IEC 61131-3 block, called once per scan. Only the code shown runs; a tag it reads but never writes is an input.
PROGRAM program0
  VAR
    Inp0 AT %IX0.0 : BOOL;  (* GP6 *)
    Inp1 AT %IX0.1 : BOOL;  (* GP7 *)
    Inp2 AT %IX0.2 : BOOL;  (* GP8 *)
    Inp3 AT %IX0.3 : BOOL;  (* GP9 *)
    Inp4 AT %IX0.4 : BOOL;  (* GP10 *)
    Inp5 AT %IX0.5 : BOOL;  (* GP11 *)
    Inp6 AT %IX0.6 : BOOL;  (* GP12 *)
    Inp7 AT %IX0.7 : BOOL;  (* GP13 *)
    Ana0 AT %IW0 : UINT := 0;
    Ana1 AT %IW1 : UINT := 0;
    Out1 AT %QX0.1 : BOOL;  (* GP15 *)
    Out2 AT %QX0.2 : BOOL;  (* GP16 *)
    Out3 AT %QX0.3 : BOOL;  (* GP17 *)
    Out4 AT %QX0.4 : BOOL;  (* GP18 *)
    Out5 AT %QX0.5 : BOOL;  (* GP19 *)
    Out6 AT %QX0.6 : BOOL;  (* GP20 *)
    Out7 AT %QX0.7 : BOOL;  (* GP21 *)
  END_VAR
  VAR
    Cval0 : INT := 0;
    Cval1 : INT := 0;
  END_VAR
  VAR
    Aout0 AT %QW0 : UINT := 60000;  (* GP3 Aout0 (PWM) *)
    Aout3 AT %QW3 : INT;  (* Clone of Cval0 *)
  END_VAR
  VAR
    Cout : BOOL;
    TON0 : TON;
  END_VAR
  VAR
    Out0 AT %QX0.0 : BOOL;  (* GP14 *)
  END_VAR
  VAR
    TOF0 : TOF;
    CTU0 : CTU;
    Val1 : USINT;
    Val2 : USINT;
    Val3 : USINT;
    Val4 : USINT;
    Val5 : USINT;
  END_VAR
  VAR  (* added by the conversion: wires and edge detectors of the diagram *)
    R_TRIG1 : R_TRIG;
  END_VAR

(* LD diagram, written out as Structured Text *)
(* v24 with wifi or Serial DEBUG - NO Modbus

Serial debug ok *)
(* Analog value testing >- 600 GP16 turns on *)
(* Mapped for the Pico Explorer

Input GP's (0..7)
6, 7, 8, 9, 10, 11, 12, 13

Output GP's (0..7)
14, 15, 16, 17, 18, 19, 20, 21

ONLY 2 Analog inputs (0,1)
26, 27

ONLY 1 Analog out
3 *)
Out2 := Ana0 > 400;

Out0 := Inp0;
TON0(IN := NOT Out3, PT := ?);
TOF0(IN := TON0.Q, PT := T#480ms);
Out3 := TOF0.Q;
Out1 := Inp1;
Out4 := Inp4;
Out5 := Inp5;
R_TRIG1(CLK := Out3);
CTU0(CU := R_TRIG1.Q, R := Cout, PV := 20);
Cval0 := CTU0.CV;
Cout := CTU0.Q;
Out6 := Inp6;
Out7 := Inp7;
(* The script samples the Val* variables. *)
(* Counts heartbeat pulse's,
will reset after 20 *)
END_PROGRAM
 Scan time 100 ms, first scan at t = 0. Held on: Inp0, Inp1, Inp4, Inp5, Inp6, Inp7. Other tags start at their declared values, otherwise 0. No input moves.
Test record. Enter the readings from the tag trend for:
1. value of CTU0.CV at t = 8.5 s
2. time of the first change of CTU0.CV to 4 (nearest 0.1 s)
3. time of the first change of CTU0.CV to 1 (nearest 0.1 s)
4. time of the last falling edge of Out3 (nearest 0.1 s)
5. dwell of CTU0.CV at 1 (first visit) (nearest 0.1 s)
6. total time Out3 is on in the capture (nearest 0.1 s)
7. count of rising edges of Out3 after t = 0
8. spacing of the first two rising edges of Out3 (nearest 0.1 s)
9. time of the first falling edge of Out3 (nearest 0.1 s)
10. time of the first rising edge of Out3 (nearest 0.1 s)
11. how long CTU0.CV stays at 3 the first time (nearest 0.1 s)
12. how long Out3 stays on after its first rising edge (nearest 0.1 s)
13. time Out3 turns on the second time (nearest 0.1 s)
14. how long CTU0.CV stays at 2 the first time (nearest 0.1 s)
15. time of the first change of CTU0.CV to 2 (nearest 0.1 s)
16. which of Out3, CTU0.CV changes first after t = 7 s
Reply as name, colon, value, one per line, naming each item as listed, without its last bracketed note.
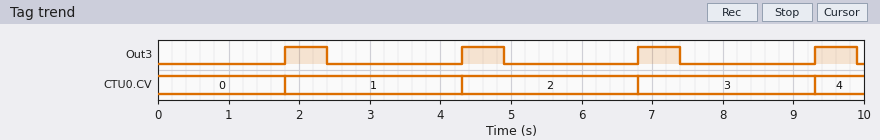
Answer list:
value of CTU0.CV at t = 8.5 s: 3
time of the first change of CTU0.CV to 4: 9.3 s
time of the first change of CTU0.CV to 1: 1.8 s
time of the last falling edge of Out3: 9.9 s
dwell of CTU0.CV at 1 (first visit): 2.5 s
total time Out3 is on in the capture: 2.4 s
count of rising edges of Out3 after t = 0: 4
spacing of the first two rising edges of Out3: 2.5 s
time of the first falling edge of Out3: 2.4 s
time of the first rising edge of Out3: 1.8 s
how long CTU0.CV stays at 3 the first time: 2.5 s
how long Out3 stays on after its first rising edge: 0.6 s
time Out3 turns on the second time: 4.3 s
how long CTU0.CV stays at 2 the first time: 2.5 s
time of the first change of CTU0.CV to 2: 4.3 s
which of Out3, CTU0.CV changes first after t = 7 s: Out3
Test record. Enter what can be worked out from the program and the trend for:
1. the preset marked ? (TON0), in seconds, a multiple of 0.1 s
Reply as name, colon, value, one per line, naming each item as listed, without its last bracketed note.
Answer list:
the preset marked ? (TON0), in seconds, a multiple of 0.1 s: 1.8 s
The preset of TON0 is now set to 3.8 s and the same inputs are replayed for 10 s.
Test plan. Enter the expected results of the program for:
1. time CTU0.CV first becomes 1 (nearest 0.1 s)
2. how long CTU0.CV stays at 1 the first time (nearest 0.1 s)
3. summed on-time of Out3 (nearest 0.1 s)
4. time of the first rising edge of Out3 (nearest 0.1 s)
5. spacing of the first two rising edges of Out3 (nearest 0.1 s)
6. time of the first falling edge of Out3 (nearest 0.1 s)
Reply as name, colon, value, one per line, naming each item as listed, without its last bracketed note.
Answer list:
time CTU0.CV first becomes 1: 3.8 s
how long CTU0.CV stays at 1 the first time: 4.5 s
summed on-time of Out3: 1.2 s
time of the first rising edge of Out3: 3.8 s
spacing of the first two rising edges of Out3: 4.5 s
time of the first falling edge of Out3: 4.4 s
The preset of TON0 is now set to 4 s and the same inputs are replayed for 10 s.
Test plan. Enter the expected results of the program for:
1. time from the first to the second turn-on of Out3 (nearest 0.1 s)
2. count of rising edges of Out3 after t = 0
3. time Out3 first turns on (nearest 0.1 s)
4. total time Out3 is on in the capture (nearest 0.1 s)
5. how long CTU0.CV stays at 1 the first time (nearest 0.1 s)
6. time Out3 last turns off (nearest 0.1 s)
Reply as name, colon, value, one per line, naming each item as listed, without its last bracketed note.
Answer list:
time from the first to the second turn-on of Out3: 4.7 s
count of rising edges of Out3 after t = 0: 2
time Out3 first turns on: 4.0 s
total time Out3 is on in the capture: 1.2 s
how long CTU0.CV stays at 1 the first time: 4.7 s
time Out3 last turns off: 9.3 s
